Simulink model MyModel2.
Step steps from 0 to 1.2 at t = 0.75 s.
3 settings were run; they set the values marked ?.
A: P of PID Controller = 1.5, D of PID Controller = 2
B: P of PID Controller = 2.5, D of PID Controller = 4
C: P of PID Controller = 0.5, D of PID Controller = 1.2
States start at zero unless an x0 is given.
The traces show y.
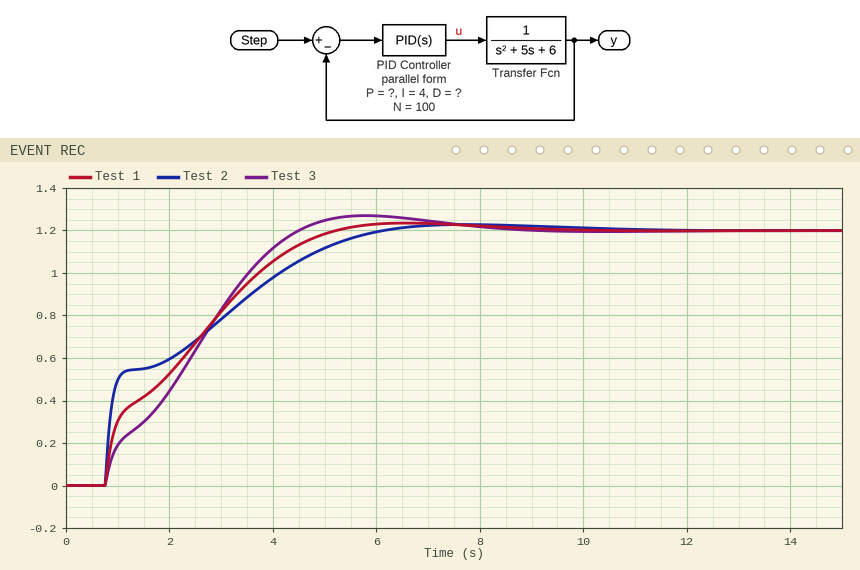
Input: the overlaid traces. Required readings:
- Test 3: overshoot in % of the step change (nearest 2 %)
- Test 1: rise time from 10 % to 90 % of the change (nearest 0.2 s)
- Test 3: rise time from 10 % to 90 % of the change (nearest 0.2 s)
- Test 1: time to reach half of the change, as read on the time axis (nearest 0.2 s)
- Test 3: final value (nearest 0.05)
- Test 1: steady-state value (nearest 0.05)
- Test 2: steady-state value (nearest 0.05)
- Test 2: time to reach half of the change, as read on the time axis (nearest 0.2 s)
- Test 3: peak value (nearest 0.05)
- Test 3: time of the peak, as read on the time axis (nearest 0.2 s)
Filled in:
6 %
3.4 s
3.0 s
2.2 s
1.20
1.20
1.20
2.0 s
1.25
5.8 s
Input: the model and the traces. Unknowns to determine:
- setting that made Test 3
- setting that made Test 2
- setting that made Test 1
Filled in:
C
B
A
